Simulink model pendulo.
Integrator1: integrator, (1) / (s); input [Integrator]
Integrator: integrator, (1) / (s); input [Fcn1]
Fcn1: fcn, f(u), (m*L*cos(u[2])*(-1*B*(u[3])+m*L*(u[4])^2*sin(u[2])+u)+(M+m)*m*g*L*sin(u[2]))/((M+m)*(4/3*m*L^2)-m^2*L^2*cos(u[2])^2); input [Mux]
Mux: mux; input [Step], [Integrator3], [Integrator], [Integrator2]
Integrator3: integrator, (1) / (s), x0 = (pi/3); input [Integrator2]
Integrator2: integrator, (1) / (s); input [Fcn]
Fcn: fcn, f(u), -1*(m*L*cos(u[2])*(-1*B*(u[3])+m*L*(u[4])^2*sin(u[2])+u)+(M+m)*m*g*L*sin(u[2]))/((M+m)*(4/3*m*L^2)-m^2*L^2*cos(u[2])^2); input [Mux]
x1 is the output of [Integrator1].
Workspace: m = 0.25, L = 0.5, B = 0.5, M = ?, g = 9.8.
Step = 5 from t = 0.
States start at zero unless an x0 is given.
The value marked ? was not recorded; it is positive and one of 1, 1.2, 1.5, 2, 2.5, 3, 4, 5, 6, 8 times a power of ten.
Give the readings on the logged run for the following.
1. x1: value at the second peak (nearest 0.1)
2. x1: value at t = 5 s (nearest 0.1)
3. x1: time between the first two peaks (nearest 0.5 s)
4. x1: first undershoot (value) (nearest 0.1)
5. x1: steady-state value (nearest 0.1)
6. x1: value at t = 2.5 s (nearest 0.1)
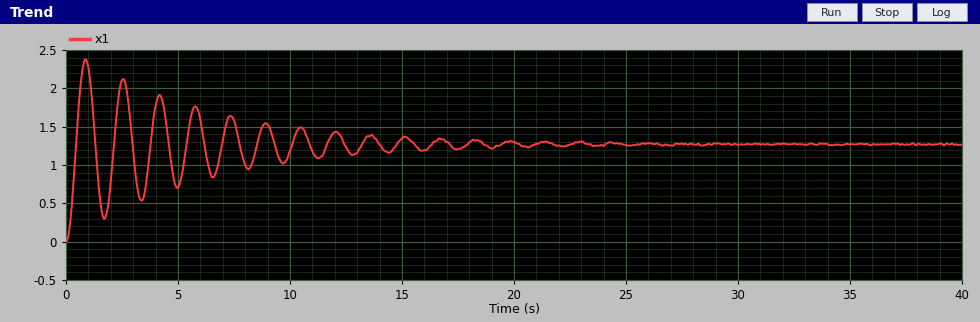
2.1
0.7
1.5 s
0.3
1.3
2.1
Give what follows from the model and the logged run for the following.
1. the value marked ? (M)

2
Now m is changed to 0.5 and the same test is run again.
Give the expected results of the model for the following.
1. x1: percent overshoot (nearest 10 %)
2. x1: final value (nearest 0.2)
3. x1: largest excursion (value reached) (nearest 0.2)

90 %
1.2
2.4
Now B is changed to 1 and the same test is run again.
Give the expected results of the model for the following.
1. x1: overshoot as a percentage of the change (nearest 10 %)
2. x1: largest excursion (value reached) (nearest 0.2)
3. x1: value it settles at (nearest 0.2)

80 %
2.2
1.2
